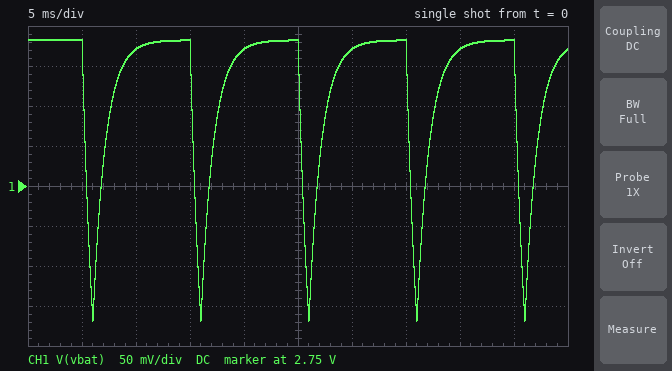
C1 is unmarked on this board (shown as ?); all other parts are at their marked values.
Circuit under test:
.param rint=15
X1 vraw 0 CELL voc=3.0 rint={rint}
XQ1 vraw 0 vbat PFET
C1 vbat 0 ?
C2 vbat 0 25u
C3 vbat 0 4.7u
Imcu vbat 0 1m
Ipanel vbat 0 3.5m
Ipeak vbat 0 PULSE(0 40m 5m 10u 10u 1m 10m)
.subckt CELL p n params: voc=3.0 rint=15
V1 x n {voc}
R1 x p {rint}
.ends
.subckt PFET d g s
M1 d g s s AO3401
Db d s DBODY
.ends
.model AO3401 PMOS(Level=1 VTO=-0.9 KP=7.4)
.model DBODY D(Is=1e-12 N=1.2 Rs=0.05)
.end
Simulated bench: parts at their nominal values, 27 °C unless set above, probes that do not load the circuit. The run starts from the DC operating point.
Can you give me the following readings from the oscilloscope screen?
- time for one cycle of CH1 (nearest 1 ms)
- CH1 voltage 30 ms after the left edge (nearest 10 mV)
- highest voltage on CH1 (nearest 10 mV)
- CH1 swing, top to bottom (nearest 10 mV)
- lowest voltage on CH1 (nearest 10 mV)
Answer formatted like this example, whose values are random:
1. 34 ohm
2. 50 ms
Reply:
1. 10 ms
2. 2.92 V
3. 2.93 V
4. 350 mV
5. 2.58 V
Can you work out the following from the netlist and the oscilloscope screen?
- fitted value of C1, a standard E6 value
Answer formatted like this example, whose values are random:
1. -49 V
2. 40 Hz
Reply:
1. 47 µF
